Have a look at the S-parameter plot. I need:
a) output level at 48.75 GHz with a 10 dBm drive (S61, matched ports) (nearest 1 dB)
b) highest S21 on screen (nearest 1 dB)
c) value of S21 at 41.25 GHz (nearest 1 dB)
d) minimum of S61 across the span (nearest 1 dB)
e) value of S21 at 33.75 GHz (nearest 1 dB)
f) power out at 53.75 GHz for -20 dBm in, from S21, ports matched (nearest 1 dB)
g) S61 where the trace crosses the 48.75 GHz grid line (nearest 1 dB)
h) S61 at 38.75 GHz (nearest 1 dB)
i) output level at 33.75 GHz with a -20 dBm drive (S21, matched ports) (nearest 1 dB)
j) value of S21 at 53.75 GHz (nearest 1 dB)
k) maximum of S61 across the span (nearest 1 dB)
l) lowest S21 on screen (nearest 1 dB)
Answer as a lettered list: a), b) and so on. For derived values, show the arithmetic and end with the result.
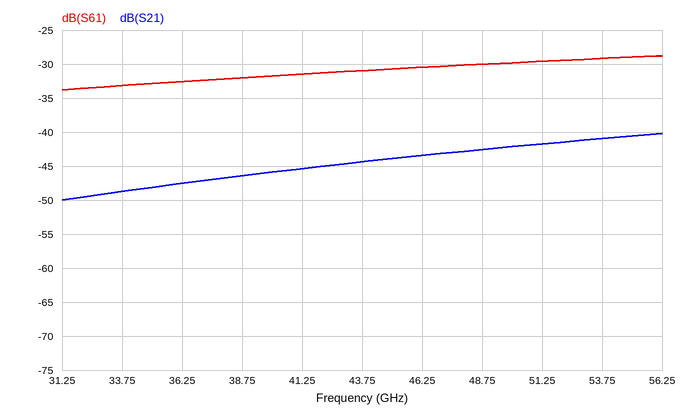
a) 10 dBm + (-30 dB) = -20 dBm
b) -40 dB
c) -45 dB
d) -34 dB
e) -49 dB
f) -20 dBm + (-41 dB) = -61 dBm
g) -30 dB
h) -32 dB
i) -20 dBm + (-49 dB) = -69 dBm
j) -41 dB
k) -29 dB
l) -50 dB
